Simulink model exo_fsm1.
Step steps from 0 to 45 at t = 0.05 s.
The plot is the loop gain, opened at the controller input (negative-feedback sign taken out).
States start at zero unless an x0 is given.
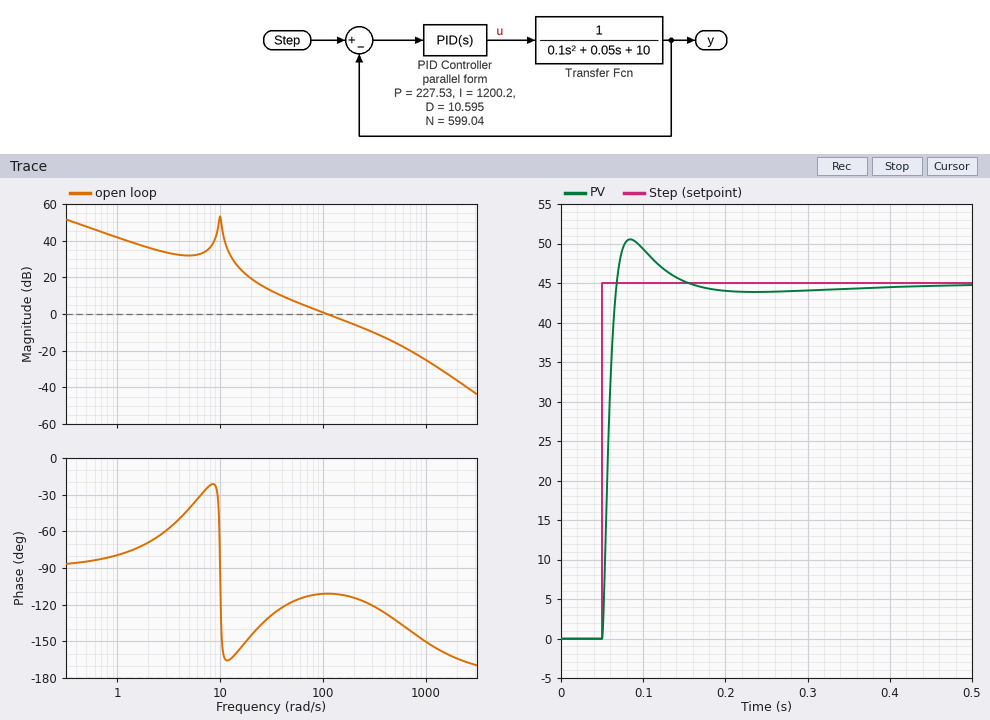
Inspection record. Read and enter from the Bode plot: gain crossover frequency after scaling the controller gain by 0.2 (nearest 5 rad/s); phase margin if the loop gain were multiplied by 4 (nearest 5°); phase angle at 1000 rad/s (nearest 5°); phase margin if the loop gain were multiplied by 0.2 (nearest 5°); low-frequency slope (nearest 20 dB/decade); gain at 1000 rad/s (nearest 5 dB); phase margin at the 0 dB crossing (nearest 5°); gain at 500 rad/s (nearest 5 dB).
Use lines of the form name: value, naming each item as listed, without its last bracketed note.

gain crossover frequency after scaling the controller gain by 0.2: 30 rad/s
phase margin if the loop gain were multiplied by 4: 55°
phase angle at 1000 rad/s: -150°
phase margin if the loop gain were multiplied by 0.2: 50°
low-frequency slope: -20 dB/decade
gain at 1000 rad/s: -25 dB
phase margin at the 0 dB crossing: 70°
gain at 500 rad/s: -15 dB
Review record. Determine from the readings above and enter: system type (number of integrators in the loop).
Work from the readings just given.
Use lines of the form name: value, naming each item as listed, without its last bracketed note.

system type: 1
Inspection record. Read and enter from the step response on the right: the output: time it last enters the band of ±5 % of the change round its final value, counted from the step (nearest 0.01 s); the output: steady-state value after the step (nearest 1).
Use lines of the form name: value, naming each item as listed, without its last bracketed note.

the output: time it last enters the band of ±5 % of the change round its final value, counted from the step: 0.07 s
the output: steady-state value after the step: 45
